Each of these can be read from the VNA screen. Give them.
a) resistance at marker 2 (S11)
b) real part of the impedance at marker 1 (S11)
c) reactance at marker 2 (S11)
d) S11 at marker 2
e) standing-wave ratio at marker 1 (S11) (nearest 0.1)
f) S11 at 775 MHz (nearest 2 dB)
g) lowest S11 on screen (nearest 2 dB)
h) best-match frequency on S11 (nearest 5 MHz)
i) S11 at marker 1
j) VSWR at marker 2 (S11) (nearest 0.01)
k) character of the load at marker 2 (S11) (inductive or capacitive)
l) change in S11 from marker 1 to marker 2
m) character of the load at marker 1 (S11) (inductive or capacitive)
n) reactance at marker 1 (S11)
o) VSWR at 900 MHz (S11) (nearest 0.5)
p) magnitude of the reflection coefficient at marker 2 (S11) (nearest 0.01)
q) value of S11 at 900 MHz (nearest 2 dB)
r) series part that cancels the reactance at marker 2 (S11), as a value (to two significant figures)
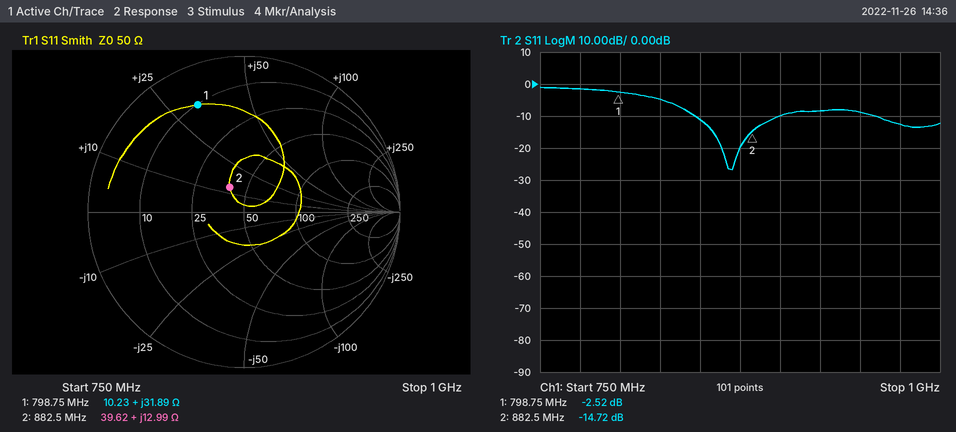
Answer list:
39.62 Ω
10.23 Ω
+12.99 Ω
-14.72 dB
6.9
-2 dB
-26 dB
870 MHz
-2.52 dB
1.45
inductive
-12.20 dB
inductive
+31.89 Ω
2.0
0.18
-10 dB
14 pF
